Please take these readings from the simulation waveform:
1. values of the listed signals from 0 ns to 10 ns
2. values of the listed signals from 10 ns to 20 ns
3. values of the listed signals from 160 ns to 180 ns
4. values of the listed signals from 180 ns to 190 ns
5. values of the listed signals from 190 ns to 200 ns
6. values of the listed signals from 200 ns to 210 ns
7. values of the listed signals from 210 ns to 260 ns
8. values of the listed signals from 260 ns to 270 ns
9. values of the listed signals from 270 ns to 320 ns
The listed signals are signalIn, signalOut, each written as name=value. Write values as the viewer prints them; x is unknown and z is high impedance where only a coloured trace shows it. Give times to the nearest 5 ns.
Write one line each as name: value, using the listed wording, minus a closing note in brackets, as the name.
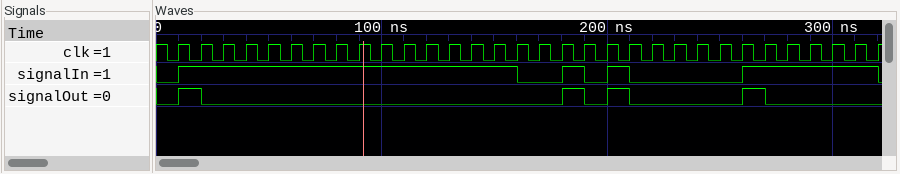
values of the listed signals from 0 ns to 10 ns: signalIn=0, signalOut=0
values of the listed signals from 10 ns to 20 ns: signalIn=1, signalOut=1
values of the listed signals from 160 ns to 180 ns: signalIn=0, signalOut=0
values of the listed signals from 180 ns to 190 ns: signalIn=1, signalOut=1
values of the listed signals from 190 ns to 200 ns: signalIn=0, signalOut=0
values of the listed signals from 200 ns to 210 ns: signalIn=1, signalOut=1
values of the listed signals from 210 ns to 260 ns: signalIn=0, signalOut=0
values of the listed signals from 260 ns to 270 ns: signalIn=1, signalOut=1
values of the listed signals from 270 ns to 320 ns: signalIn=1, signalOut=0
